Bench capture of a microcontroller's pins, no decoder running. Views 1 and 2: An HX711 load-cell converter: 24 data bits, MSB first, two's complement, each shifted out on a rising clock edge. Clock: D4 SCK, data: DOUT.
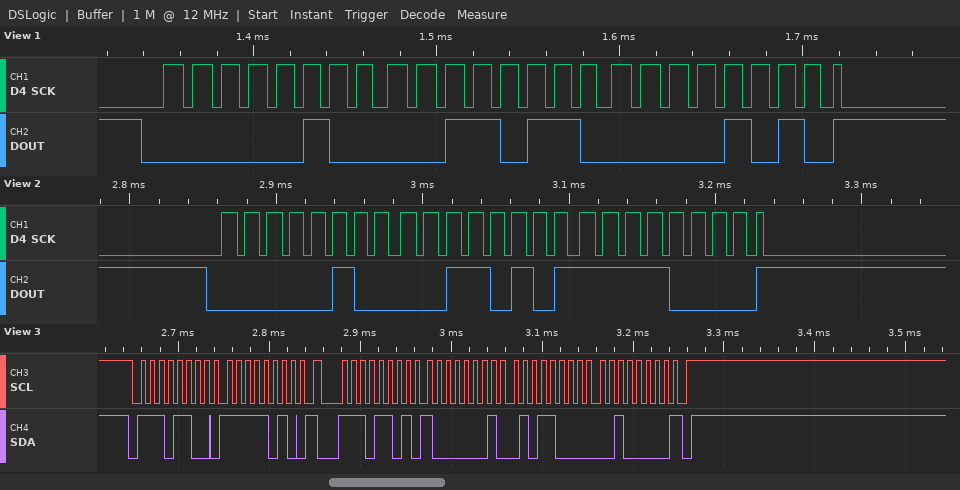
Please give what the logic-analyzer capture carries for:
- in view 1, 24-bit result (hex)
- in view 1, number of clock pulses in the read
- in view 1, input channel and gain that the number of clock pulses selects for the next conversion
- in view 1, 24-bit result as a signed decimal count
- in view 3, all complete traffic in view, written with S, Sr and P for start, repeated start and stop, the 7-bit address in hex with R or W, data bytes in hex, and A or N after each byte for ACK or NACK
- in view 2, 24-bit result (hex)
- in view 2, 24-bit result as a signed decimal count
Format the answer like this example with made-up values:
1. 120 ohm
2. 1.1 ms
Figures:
1. 0x04360A
2. 25
3. channel A, gain 128
4. 275978
5. S 76W A FA A Sr 76R A 81 A 58 A 20 N P
6. 0x0435F0
7. 275952
